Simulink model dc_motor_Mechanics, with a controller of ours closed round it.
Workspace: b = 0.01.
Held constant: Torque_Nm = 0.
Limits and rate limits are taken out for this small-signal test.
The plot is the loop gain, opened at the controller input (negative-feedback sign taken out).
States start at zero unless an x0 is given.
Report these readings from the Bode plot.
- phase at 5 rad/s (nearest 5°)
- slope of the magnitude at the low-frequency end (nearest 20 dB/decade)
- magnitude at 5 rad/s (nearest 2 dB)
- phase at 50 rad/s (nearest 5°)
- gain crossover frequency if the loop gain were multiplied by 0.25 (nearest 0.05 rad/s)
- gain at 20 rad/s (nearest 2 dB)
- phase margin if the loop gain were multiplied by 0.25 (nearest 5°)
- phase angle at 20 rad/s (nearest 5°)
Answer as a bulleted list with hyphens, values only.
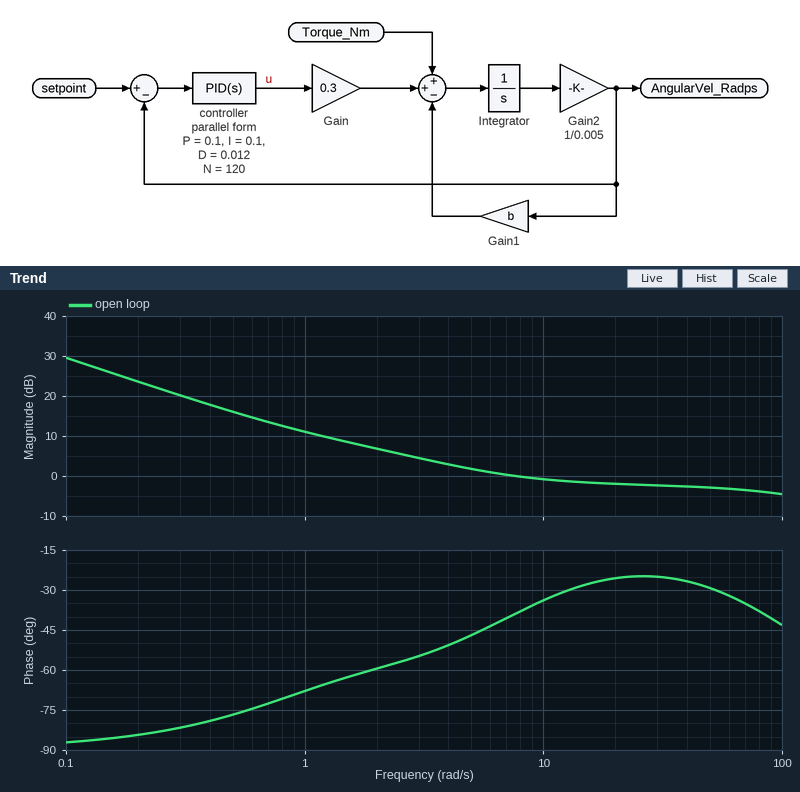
- -45°
- -20 dB/decade
- 2 dB
- -30°
- 0.85 rad/s
- -2 dB
- 110°
- -25°
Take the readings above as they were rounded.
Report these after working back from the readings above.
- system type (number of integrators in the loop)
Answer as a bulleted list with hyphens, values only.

- 1
